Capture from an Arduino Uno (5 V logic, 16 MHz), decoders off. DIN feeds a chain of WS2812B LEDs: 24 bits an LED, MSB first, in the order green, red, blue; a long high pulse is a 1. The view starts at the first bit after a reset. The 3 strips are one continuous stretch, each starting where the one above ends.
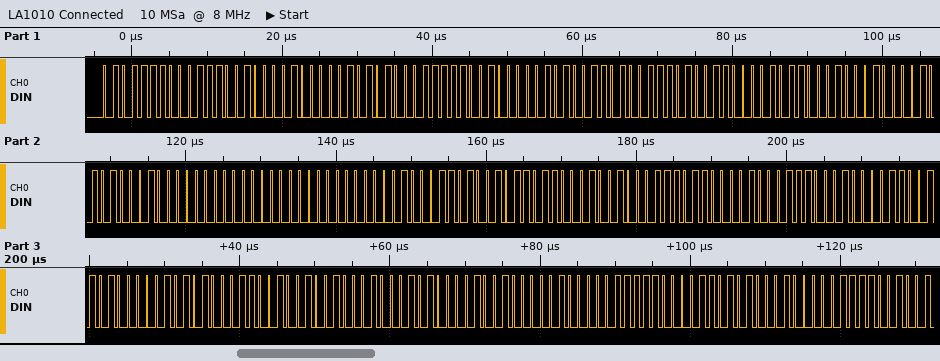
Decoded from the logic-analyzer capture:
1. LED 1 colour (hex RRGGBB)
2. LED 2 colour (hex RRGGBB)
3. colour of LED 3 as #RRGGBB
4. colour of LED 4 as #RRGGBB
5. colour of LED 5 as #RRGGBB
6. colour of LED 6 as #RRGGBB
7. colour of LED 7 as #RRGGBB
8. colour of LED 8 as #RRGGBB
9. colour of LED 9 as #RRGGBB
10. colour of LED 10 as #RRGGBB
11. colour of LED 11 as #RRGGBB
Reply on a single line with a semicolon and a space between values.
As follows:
#395E08; #3E2A41; #3A4D61; #216251; #000000; #4B2362; #61471C; #344315; #241945; #04091F; #440D1E
